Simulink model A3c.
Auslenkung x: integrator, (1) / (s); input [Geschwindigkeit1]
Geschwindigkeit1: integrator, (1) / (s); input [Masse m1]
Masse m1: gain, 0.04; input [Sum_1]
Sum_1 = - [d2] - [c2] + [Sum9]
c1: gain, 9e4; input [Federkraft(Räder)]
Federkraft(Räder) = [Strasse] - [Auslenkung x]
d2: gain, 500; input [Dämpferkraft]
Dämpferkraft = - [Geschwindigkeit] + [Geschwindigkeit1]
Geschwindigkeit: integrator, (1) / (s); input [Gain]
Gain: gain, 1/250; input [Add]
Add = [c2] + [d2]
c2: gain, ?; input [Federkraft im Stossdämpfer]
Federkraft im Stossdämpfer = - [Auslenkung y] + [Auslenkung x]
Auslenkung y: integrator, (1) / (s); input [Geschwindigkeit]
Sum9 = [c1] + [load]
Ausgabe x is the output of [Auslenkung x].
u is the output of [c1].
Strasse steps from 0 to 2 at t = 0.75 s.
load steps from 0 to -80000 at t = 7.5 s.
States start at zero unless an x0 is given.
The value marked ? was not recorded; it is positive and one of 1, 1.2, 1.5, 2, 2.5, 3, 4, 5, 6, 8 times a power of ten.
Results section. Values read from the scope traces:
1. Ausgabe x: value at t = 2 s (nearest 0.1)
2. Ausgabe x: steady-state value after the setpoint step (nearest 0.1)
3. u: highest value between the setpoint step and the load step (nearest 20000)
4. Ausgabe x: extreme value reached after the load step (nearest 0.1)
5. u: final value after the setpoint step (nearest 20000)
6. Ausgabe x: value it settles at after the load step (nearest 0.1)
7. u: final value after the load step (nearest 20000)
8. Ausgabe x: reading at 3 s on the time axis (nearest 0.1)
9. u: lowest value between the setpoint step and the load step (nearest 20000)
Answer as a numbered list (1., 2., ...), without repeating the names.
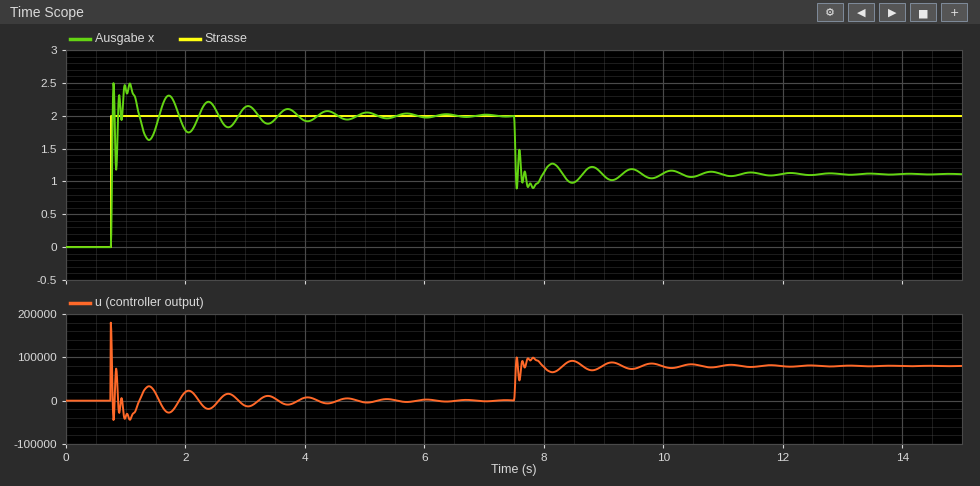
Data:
1. 1.8
2. 2.0
3. 180000
4. 0.9
5. 0
6. 1.1
7. 80000
8. 2.1
9. -40000
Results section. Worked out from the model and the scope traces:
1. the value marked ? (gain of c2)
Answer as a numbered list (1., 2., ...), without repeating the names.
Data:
1. 30000
